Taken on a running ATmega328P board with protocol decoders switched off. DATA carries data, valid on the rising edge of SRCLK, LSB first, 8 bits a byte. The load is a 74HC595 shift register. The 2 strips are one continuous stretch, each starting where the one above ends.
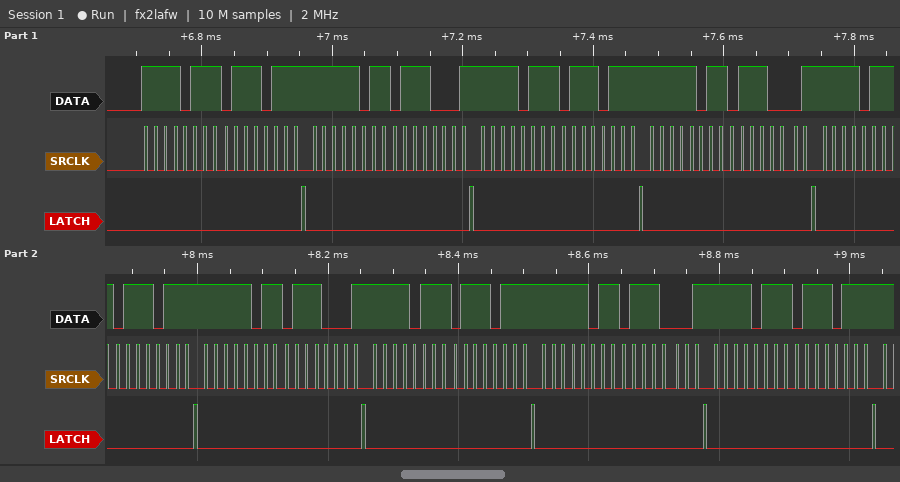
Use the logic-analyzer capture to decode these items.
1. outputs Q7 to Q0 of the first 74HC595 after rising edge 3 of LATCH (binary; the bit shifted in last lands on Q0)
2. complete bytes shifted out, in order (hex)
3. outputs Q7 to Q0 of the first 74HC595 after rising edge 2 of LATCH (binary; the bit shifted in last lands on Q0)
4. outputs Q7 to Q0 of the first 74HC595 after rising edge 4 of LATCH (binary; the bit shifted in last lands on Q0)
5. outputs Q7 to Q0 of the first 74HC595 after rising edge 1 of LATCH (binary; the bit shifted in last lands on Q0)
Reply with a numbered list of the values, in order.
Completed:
1. 01110111
2. 0xEF 0xEE 0xDF 0x8E 0xEF 0xEE 0xDF 0x8E 0xEF 0xEE 0xDF 0x8E 0xEF 0xEE 0xDF 0x8E 0xEF 0xEE
3. 01110001
4. 01110001
5. 01110111
